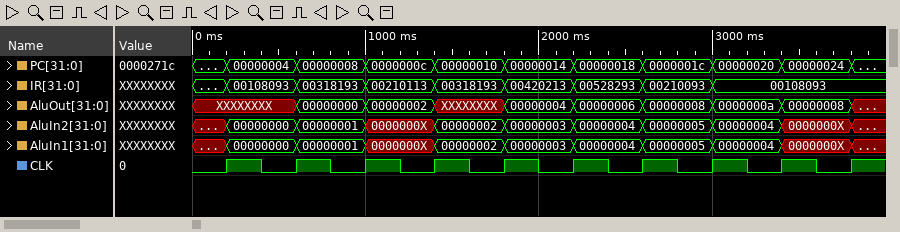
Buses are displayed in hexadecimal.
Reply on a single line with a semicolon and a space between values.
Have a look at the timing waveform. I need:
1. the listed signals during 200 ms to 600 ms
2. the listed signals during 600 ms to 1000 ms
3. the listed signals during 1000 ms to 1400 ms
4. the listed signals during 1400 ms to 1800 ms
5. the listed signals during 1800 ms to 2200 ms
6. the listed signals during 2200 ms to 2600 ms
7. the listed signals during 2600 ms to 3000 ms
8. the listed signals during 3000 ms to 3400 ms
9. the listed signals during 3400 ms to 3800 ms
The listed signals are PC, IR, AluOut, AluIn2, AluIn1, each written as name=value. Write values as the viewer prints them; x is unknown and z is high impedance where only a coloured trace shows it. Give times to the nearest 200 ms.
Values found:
PC=00000004, IR=00108093, AluOut=XXXXXXXX, AluIn2=00000000, AluIn1=00000000; PC=00000008, IR=00318193, AluOut=00000000, AluIn2=00000001, AluIn1=00000001; PC=0000000c, IR=00210113, AluOut=00000002, AluIn2=0000000X, AluIn1=0000000X; PC=00000010, IR=00318193, AluOut=XXXXXXXX, AluIn2=00000002, AluIn1=00000002; PC=00000014, IR=00420213, AluOut=00000004, AluIn2=00000003, AluIn1=00000003; PC=00000018, IR=00528293, AluOut=00000006, AluIn2=00000004, AluIn1=00000004; PC=0000001c, IR=00210093, AluOut=00000008, AluIn2=00000005, AluIn1=00000005; PC=00000020, IR=00108093, AluOut=0000000a, AluIn2=00000004, AluIn1=00000004; PC=00000024, IR=00108093, AluOut=00000008, AluIn2=0000000X, AluIn1=0000000X
